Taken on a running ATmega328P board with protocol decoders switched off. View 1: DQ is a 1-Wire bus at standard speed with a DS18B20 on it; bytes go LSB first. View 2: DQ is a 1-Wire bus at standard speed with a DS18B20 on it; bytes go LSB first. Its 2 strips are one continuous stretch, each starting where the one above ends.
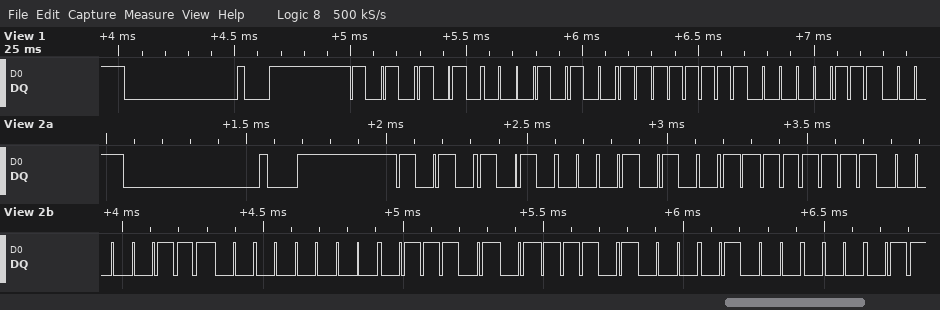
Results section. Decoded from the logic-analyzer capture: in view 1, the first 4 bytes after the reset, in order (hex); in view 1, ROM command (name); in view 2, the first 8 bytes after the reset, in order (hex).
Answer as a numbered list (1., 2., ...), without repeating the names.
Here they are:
1. 55 28 FF E0
2. Match ROM
3. 55 28 FF E0 00 AE 17 02
